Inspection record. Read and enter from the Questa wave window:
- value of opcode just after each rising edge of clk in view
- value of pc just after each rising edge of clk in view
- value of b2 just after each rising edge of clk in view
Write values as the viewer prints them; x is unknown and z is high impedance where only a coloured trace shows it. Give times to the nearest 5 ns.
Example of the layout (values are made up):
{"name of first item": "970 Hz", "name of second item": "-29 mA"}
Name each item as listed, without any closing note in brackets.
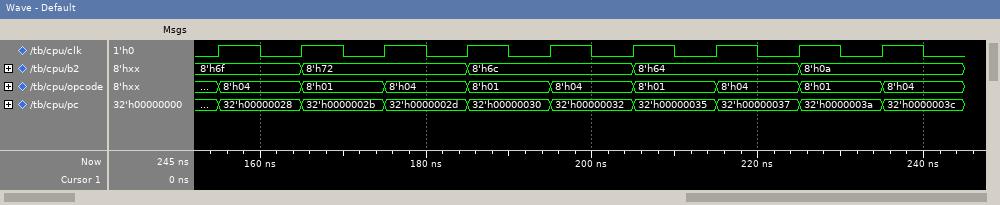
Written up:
{"value of opcode just after each rising edge of clk in view": "8'h04, 8'h01, 8'h04, 8'h01, 8'h04, 8'h01, 8'h04, 8'h01, 8'h04", "value of pc just after each rising edge of clk in view": "32'h00000028, 32'h0000002b, 32'h0000002d, 32'h00000030, 32'h00000032, 32'h00000035, 32'h00000037, 32'h0000003a, 32'h0000003c", "value of b2 just after each rising edge of clk in view": "8'h6f, 8'h72, 8'h72, 8'h6c, 8'h6c, 8'h64, 8'h64, 8'h0a, 8'h0a"}
